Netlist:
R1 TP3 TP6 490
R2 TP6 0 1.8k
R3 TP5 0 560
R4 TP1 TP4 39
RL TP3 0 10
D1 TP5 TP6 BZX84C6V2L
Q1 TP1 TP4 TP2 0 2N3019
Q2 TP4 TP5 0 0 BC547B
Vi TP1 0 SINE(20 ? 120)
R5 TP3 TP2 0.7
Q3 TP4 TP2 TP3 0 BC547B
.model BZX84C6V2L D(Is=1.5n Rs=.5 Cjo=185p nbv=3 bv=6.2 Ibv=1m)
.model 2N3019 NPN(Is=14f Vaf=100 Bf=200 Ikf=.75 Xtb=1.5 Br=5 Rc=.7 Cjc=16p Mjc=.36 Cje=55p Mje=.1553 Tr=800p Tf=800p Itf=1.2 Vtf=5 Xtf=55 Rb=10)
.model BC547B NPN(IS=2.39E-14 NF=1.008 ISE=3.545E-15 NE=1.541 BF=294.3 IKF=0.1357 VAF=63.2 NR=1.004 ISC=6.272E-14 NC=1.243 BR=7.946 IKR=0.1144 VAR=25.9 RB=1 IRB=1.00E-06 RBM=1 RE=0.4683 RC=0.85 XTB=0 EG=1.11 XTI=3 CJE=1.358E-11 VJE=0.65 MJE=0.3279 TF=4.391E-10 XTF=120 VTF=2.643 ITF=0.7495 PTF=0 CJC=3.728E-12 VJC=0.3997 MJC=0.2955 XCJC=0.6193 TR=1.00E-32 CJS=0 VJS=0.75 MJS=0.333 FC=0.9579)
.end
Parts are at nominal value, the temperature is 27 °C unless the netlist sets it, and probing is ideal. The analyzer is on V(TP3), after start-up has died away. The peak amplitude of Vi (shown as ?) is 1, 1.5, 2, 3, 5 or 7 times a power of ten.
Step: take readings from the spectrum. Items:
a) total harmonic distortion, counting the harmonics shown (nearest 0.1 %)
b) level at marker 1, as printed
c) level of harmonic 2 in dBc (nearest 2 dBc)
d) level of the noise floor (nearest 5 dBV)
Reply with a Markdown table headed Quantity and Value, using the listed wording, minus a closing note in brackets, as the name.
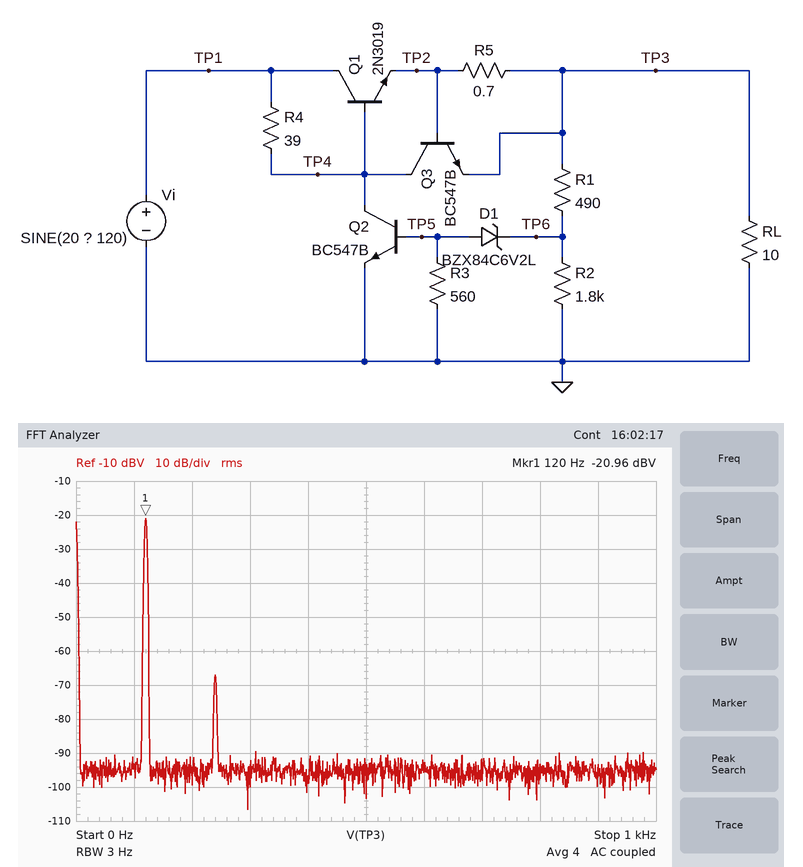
| Quantity | Value |
|---|---|
| total harmonic distortion, counting the harmonics shown | 0.5 % |
| level at marker 1, as printed | -20.96 dBV |
| level of harmonic 2 in dBc | -46 dBc |
| level of the noise floor | -95 dBV |
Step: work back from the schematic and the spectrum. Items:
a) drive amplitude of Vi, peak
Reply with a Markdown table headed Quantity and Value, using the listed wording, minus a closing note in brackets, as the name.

| Quantity | Value |
|---|---|
| drive amplitude of Vi, peak | 1 V |
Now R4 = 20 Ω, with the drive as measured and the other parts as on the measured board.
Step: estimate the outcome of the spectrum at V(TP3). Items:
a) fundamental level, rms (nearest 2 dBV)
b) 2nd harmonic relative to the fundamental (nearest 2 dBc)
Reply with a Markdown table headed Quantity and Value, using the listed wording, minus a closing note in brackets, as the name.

| Quantity | Value |
|---|---|
| fundamental level, rms | -16 dBV |
| 2nd harmonic relative to the fundamental | -48 dBc |
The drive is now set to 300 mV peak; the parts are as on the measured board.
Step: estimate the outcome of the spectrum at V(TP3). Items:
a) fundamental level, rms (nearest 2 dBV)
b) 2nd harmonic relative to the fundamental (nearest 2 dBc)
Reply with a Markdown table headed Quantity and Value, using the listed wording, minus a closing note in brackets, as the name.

| Quantity | Value |
|---|---|
| fundamental level, rms | -32 dBV |
| 2nd harmonic relative to the fundamental | -56 dBc |
